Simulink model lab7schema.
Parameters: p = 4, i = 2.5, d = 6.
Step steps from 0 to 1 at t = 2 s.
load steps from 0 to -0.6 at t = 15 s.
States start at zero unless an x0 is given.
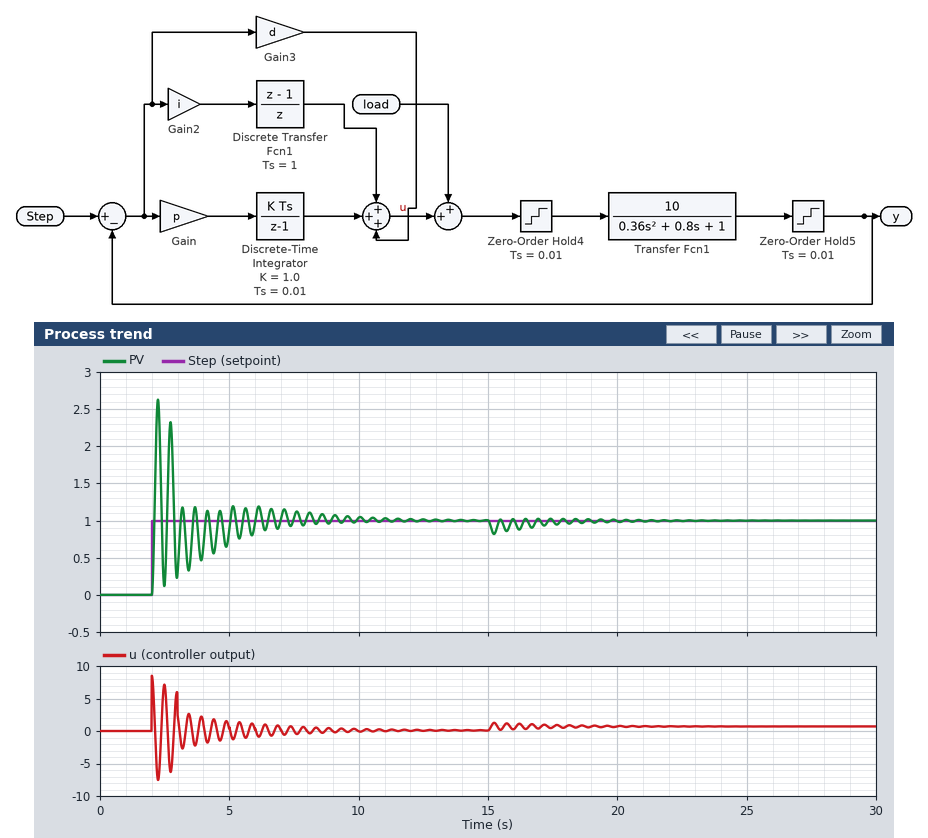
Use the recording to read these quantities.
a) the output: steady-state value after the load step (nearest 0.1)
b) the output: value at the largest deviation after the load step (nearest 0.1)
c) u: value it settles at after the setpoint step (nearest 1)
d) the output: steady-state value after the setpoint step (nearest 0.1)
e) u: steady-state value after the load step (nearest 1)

1.0
0.8
0
1.0
1
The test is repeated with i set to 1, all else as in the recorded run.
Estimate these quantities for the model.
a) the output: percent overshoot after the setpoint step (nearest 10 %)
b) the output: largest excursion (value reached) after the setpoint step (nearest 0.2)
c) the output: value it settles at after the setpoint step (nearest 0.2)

120 %
2.2
1.0
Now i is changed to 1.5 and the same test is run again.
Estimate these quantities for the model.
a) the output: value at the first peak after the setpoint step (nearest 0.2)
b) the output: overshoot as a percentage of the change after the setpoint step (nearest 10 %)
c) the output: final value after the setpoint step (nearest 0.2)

2.4
130 %
1.0
